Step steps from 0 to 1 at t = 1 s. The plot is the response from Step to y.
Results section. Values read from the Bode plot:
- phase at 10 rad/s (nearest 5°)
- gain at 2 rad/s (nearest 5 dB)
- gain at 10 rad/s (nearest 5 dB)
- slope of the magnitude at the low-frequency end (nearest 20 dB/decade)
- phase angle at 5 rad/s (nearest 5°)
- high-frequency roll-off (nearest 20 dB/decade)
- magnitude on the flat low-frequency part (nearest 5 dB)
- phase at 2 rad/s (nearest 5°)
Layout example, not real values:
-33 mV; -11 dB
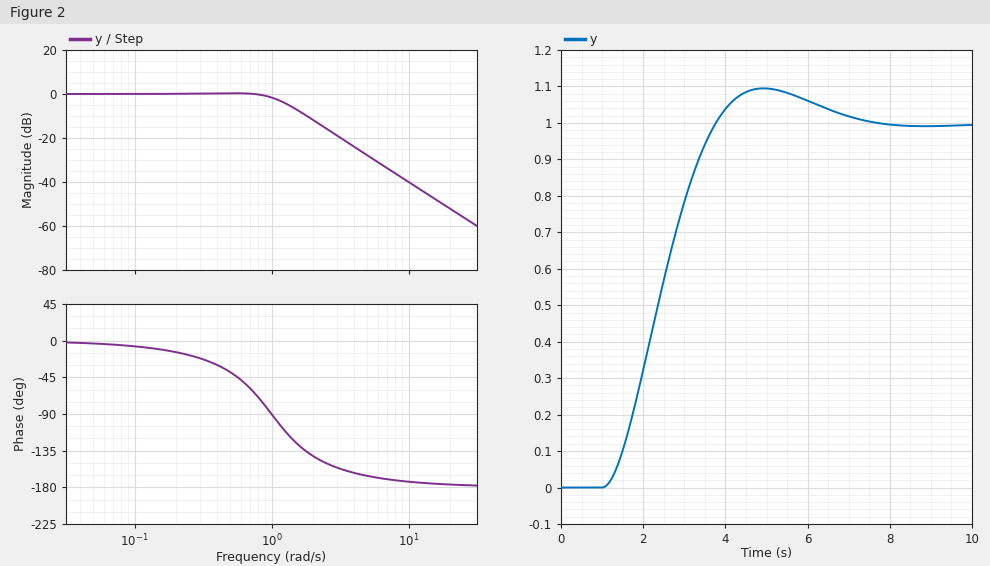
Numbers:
-175°; -10 dB; -40 dB; 0 dB/decade; -165°; -40 dB/decade; 0 dB; -140°
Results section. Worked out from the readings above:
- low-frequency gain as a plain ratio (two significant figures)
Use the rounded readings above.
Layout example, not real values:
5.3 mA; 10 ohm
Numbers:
1.0
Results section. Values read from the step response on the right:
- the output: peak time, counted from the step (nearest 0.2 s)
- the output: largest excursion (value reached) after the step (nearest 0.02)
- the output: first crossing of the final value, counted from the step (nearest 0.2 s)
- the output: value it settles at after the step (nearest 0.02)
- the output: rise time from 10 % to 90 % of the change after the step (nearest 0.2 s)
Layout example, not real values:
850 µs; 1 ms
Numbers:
4.0 s; 1.10; 2.8 s; 1.00; 1.8 s
